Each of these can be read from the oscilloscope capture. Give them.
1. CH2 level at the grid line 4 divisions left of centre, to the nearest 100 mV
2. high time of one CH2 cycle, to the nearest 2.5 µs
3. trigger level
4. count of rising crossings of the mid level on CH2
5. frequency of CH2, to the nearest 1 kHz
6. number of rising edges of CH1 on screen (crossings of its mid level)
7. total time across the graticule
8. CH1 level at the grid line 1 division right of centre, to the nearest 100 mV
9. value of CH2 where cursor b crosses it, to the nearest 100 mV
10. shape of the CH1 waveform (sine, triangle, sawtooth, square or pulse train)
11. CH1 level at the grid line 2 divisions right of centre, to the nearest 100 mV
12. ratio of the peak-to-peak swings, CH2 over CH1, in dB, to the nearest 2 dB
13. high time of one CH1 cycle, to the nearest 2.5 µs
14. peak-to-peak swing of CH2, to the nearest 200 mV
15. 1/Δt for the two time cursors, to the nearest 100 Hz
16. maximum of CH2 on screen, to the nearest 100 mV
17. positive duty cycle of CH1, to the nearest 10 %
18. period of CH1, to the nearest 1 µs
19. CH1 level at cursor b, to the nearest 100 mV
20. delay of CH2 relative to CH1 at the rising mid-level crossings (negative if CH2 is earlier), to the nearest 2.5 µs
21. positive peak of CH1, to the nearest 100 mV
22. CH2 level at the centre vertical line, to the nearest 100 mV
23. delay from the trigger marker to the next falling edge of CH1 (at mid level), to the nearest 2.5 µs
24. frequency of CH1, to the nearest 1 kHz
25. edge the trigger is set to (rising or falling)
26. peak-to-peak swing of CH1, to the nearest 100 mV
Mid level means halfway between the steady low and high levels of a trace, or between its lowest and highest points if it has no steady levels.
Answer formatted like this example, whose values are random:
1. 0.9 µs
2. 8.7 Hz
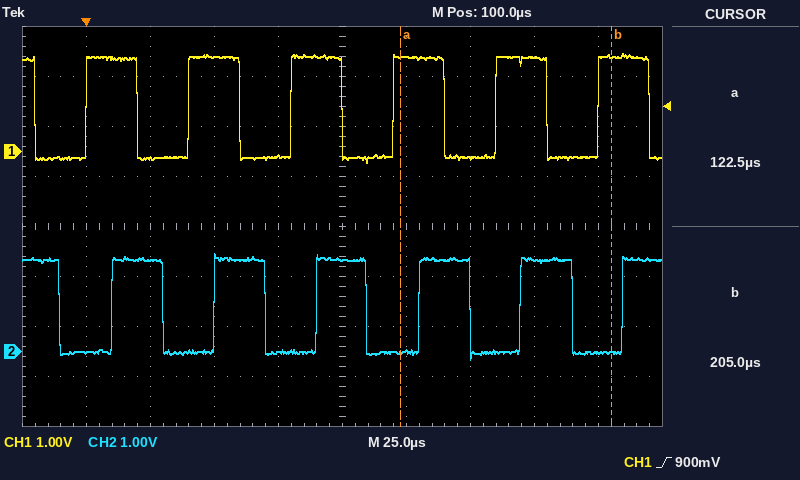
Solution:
1. 0.0 V
2. 20.0 µs
3. 900 mV
4. 6
5. 25 kHz
6. 6
7. 250 µs
8. 1.9 V
9. 0.0 V
10. square
11. -100 mV
12. 0 dB
13. 20.0 µs
14. 2.2 V
15. 12.1 kHz
16. 2.0 V
17. 50 %
18. 40 µs
19. 1.9 V
20. +10.0 µs
21. 2.0 V
22. 1.8 V
23. 20.0 µs
24. 25 kHz
25. rising
26. 2.2 V
